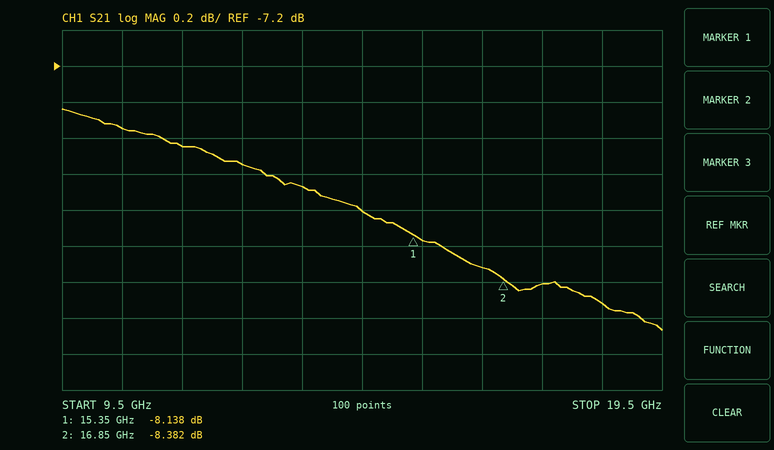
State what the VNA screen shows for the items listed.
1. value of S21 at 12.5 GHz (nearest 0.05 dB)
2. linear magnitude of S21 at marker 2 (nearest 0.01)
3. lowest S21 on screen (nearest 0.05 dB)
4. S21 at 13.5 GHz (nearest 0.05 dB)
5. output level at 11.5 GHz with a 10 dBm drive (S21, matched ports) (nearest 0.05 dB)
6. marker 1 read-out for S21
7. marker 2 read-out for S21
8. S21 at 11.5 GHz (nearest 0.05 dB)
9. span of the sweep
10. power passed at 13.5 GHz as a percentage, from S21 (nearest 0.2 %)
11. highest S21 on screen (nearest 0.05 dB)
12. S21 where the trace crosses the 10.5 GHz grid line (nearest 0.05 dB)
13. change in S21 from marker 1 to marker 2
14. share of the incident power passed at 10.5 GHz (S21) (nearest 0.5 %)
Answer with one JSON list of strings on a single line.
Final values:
["-7.75 dB", "0.38", "-8.65 dB", "-7.85 dB", "2.35 dBm", "-8.138 dB", "-8.382 dB", "-7.65 dB", "10 GHz", "16.4 %", "-7.45 dB", "-7.55 dB", "-0.244 dB", "17.5 %"]
